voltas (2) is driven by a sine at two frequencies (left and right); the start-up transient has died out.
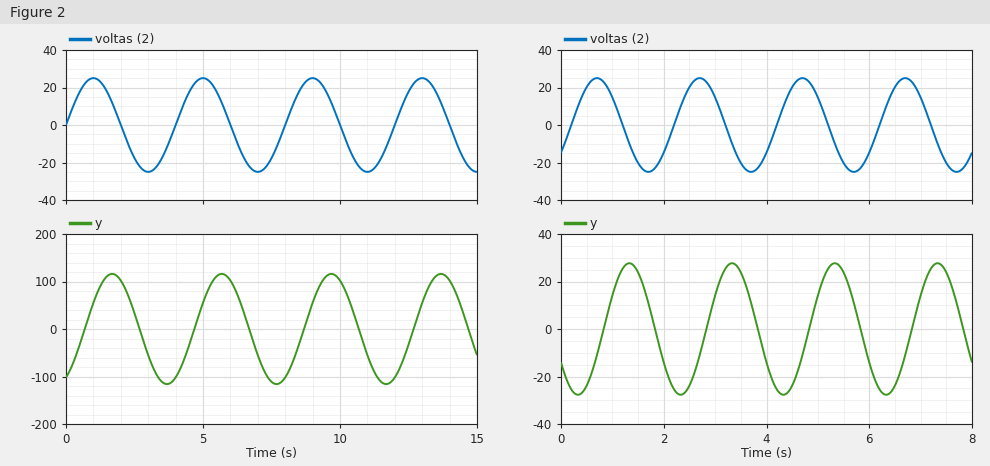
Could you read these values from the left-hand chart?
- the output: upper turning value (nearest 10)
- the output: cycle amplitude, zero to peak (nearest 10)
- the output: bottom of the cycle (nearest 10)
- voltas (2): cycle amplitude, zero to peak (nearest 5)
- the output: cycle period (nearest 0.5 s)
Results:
120
120
-120
25
4.0 s
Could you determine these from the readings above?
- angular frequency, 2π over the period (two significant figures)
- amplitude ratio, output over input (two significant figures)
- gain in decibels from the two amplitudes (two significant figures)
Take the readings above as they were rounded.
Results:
1.6 rad/s
4.8
14 dB
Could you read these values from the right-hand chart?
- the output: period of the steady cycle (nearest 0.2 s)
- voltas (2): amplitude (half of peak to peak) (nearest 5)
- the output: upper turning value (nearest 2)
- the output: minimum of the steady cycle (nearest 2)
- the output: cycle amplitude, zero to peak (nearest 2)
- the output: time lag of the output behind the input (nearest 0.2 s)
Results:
2.0 s
25
28
-28
28
0.6 s
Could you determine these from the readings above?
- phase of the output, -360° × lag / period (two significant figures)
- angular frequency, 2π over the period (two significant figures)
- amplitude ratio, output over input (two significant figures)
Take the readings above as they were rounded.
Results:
-110°
3.1 rad/s
1.1
